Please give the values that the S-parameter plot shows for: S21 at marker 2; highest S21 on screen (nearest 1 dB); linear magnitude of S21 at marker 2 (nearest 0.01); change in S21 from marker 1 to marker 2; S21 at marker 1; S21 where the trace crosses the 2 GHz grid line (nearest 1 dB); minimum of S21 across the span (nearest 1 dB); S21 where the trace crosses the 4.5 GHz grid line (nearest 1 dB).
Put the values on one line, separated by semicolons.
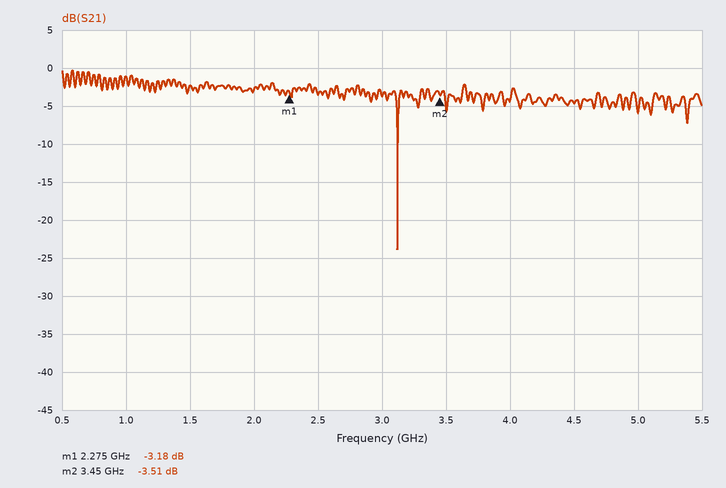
-3.51 dB; 0 dB; 0.67; -0.33 dB; -3.18 dB; -3 dB; -24 dB; -5 dB
